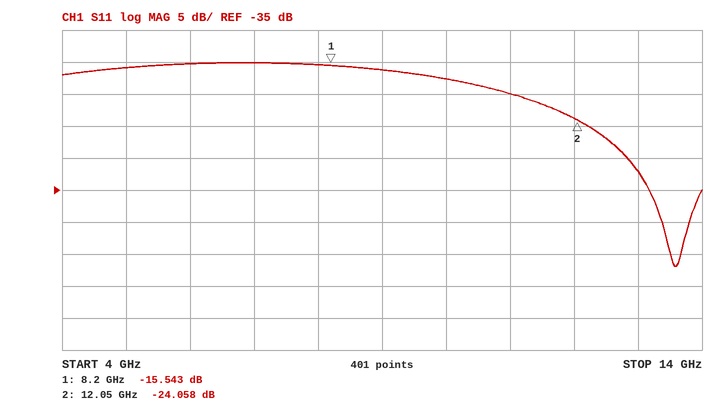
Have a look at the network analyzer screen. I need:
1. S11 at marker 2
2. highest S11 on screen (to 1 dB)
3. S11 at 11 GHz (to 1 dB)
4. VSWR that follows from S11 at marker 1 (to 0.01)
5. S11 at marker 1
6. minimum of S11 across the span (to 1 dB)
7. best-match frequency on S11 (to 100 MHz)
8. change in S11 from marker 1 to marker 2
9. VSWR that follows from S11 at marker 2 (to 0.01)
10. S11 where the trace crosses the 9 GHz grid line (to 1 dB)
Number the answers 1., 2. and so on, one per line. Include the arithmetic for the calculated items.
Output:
1. -24.058 dB
2. -15 dB
3. -20 dB
4. (1 + 0.1671)/(1 − 0.1671) ≈ 1.40
5. -15.543 dB
6. -47 dB
7. 13.6 GHz
8. -24.058 − (-15.543) = -8.515 dB
9. (1 + 0.0627)/(1 − 0.0627) ≈ 1.13
10. -16 dB
